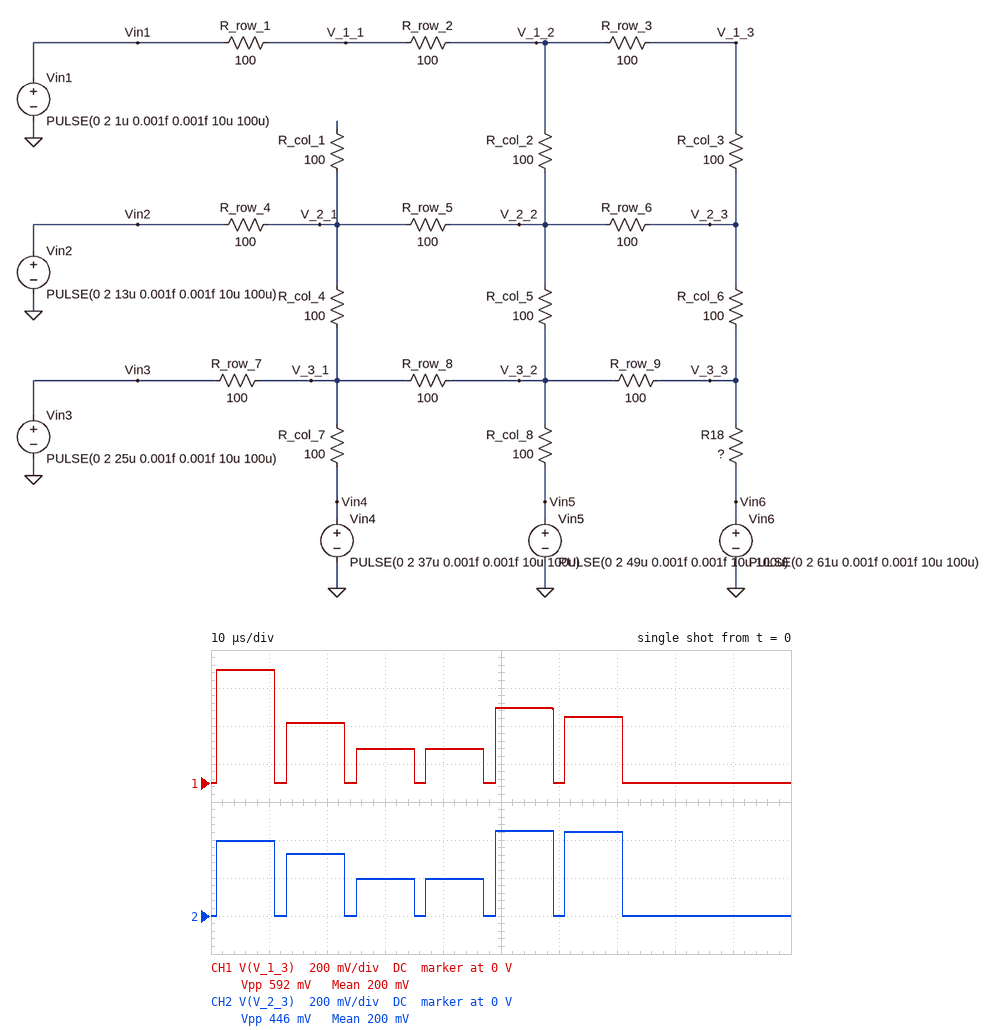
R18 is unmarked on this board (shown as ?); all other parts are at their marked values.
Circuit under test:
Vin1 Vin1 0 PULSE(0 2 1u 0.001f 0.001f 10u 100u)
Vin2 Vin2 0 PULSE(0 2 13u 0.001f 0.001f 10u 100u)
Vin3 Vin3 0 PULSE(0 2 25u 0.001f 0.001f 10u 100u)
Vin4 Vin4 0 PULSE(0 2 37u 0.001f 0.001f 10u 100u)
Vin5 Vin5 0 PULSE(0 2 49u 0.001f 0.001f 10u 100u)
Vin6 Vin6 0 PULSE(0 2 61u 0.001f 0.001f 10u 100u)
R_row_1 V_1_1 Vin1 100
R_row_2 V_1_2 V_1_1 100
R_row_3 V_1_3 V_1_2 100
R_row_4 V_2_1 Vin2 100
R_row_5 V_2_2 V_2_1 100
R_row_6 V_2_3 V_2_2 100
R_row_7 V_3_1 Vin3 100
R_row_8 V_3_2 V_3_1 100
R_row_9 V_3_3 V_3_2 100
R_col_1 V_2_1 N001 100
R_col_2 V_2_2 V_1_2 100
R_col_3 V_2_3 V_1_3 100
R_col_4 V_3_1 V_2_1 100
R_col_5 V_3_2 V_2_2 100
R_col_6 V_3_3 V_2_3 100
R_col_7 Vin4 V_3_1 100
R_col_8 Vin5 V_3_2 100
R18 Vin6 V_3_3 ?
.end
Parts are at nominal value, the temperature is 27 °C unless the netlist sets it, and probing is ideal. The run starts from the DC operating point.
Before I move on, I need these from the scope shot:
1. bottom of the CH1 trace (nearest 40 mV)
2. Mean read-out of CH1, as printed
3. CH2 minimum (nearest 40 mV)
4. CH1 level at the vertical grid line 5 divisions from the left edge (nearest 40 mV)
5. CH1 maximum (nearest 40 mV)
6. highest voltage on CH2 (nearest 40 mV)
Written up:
0 V
200 mV
0 V
400 mV
600 mV
440 mV
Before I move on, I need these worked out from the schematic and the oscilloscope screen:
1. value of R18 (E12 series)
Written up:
180 Ω
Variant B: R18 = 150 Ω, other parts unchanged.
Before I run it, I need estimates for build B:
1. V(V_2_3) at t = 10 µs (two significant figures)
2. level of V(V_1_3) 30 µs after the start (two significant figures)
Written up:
390 mV
170 mV
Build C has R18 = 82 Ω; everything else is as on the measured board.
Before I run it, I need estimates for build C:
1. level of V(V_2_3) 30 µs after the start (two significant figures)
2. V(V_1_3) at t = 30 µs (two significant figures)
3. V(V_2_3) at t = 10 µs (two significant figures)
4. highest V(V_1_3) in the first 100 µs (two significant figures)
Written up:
160 mV
150 mV
360 mV
560 mV
